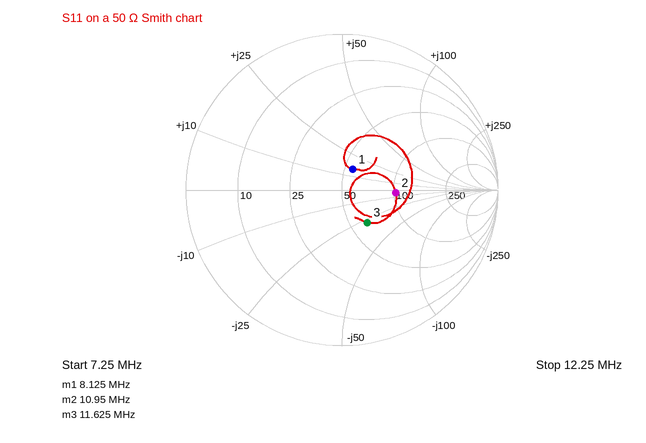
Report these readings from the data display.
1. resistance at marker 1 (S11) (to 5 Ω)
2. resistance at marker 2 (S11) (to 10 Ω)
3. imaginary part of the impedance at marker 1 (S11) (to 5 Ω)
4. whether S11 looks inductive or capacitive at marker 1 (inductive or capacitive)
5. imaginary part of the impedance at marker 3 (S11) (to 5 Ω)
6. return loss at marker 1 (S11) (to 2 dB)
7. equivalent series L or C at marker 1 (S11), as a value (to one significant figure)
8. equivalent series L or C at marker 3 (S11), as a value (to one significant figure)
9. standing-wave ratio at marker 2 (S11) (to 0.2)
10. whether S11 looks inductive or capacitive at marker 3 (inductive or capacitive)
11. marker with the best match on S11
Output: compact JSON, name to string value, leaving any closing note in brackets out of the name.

{"resistance at marker 1 (S11)": "55 Ω", "resistance at marker 2 (S11)": "100 Ω", "imaginary part of the impedance at marker 1 (S11)": "+15 Ω", "whether S11 looks inductive or capacitive at marker 1": "inductive", "imaginary part of the impedance at marker 3 (S11)": "-30 Ω", "return loss at marker 1 (S11)": "16 dB", "equivalent series L or C at marker 1 (S11), as a value": "300 nH", "equivalent series L or C at marker 3 (S11), as a value": "500 pF", "standing-wave ratio at marker 2 (S11)": "2.0", "whether S11 looks inductive or capacitive at marker 3": "capacitive", "marker with the best match on S11": "marker 1"}
